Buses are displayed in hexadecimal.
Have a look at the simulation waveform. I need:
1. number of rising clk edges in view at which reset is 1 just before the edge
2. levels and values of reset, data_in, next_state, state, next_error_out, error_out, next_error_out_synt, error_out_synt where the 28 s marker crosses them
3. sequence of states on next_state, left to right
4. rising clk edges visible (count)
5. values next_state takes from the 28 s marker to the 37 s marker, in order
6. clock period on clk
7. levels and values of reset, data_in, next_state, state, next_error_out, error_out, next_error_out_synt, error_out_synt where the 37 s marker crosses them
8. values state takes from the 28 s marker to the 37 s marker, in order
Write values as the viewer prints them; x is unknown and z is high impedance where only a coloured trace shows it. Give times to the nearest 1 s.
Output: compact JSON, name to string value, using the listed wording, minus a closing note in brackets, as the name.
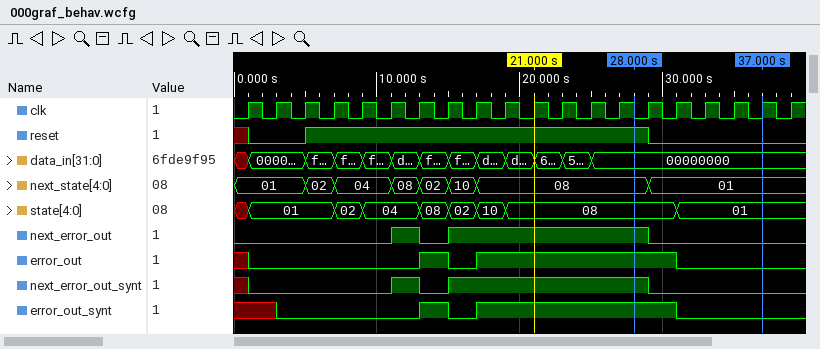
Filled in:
{"number of rising clk edges in view at which reset is 1 just before the edge": "12", "levels and values of reset, data_in, next_state, state, next_error_out, error_out, next_error_out_synt, error_out_synt where the 28 s marker crosses them": "reset=1, data_in=00000000, next_state=08, state=08, next_error_out=1, error_out=1, next_error_out_synt=1, error_out_synt=1", "sequence of states on next_state, left to right": "01, 02, 04, 08, 02, 10, 08, 01", "rising clk edges visible": "20", "values next_state takes from the 28 s marker to the 37 s marker, in order": "08, 01", "clock period on clk": "2 s", "levels and values of reset, data_in, next_state, state, next_error_out, error_out, next_error_out_synt, error_out_synt where the 37 s marker crosses them": "reset=0, data_in=00000000, next_state=01, state=01, next_error_out=0, error_out=0, next_error_out_synt=0, error_out_synt=0", "values state takes from the 28 s marker to the 37 s marker, in order": "08, 01"}
